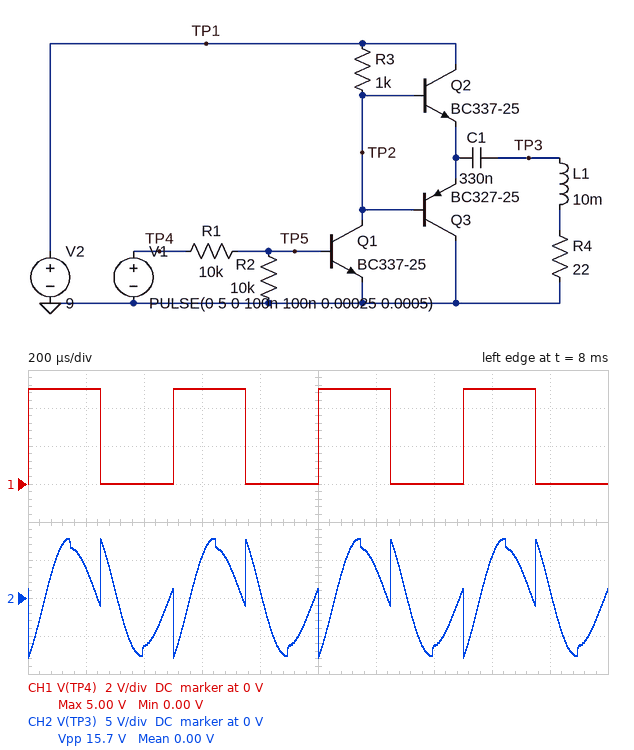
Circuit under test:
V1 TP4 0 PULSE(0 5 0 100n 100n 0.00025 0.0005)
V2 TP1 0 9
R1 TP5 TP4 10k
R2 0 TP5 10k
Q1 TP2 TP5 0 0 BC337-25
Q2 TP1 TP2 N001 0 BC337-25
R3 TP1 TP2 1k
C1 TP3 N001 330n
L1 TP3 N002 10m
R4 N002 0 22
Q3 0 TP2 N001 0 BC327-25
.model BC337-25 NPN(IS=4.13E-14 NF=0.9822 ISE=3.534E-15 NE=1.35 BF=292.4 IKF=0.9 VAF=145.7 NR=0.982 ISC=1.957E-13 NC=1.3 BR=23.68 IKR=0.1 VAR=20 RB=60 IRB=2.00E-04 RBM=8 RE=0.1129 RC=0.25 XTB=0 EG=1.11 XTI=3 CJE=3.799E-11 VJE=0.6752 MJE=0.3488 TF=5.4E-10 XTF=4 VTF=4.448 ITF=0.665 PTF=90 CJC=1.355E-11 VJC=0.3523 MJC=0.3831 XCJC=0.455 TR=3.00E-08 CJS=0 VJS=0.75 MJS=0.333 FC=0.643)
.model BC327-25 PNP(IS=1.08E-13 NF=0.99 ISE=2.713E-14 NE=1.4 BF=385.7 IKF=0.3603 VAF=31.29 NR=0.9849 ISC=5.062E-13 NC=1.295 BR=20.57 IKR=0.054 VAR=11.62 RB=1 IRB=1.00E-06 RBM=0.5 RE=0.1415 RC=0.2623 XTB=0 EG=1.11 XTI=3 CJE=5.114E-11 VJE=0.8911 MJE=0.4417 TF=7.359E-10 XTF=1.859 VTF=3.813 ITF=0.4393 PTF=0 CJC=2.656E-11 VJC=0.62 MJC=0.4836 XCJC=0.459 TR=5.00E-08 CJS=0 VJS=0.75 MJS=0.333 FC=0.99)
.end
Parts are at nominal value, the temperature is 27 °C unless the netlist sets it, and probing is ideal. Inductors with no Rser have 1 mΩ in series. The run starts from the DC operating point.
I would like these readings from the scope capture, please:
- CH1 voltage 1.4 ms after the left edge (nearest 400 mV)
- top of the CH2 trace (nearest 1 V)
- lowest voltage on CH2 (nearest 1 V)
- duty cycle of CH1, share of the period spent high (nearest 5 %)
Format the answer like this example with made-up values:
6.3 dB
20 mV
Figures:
0 V
8 V
-8 V
50 %
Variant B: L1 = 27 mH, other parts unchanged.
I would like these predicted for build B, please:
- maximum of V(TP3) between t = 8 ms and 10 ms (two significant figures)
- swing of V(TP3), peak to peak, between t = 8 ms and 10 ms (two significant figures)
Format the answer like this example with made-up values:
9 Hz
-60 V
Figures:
18 V
36 V
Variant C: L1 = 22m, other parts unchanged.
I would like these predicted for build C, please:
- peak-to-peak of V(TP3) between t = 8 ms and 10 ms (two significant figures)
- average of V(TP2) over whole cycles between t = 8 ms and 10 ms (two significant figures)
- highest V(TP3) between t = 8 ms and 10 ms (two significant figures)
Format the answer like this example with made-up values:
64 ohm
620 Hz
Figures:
68 V
4.4 V
34 V
